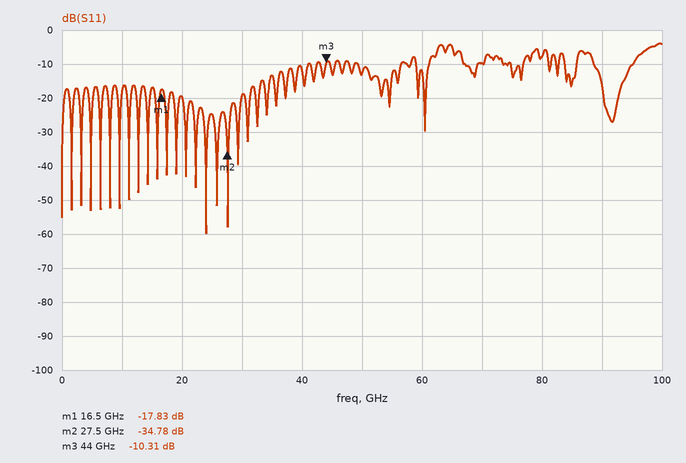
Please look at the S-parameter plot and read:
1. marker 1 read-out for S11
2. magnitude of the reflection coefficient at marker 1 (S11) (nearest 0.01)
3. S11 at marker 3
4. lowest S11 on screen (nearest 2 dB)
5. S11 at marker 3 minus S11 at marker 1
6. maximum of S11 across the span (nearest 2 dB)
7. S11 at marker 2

-17.83 dB
0.13
-10.31 dB
-60 dB
7.52 dB
-4 dB
-34.78 dB
